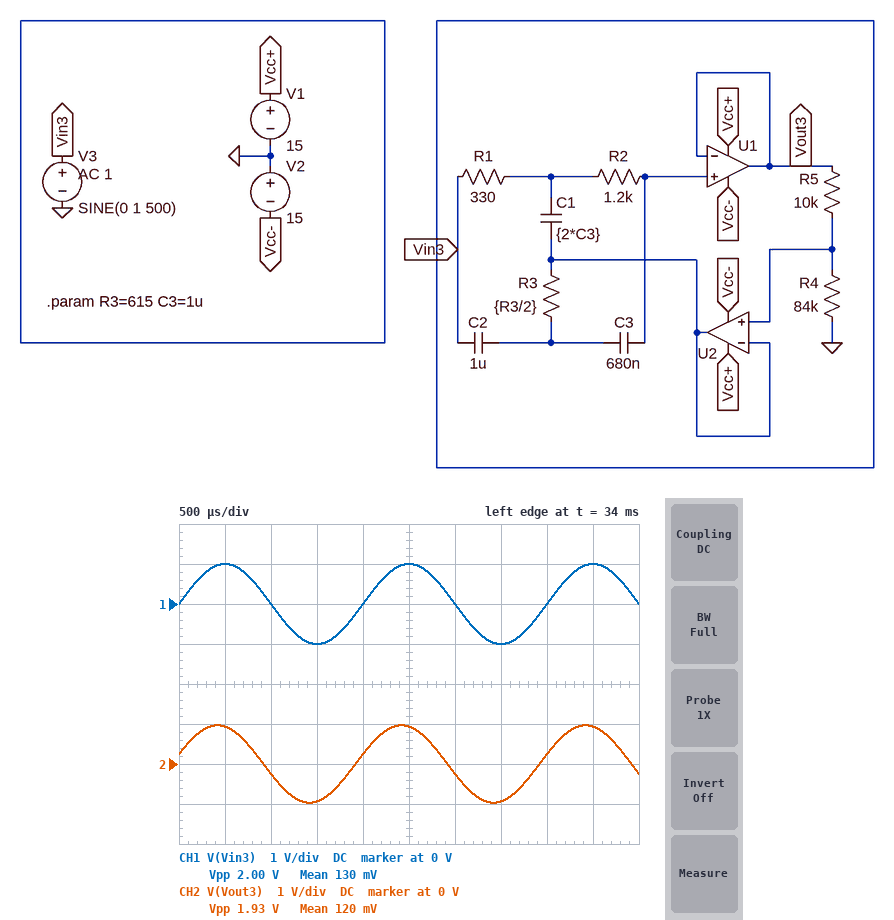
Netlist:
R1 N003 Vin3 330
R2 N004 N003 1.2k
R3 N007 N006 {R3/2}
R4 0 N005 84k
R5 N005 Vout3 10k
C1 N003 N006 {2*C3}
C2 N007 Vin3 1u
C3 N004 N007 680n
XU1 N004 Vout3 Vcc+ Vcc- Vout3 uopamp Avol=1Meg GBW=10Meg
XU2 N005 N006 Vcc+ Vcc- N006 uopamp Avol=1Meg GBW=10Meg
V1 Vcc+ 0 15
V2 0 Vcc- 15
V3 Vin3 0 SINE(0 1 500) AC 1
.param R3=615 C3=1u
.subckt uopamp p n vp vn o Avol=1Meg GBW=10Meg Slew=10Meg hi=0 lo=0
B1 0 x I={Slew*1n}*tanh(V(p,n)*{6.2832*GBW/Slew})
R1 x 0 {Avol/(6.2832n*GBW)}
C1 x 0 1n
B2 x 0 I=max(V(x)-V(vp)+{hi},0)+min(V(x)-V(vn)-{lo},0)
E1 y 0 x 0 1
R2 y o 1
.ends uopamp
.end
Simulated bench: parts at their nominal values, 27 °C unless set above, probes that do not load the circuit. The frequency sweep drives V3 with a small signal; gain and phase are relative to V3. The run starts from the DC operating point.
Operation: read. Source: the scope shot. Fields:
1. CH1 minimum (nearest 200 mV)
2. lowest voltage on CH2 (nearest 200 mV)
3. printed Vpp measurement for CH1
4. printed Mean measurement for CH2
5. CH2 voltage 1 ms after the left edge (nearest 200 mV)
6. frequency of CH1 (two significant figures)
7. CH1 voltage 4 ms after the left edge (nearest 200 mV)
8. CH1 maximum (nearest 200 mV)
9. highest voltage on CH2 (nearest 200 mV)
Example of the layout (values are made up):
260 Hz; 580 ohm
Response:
-1.0 V; -1.0 V; 2.00 V; 120 mV; -200 mV; 500 Hz; 0 V; 1.0 V; 1.0 V
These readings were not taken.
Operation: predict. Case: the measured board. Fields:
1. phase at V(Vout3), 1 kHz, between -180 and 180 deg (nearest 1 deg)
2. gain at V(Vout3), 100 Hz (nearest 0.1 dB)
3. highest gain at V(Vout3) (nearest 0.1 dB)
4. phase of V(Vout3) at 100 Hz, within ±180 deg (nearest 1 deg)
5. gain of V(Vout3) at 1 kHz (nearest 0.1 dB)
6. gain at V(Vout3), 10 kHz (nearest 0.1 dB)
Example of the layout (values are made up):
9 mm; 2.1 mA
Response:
6 deg; -0.1 dB; 0 dB; -7 deg; 0 dB; 0 dB
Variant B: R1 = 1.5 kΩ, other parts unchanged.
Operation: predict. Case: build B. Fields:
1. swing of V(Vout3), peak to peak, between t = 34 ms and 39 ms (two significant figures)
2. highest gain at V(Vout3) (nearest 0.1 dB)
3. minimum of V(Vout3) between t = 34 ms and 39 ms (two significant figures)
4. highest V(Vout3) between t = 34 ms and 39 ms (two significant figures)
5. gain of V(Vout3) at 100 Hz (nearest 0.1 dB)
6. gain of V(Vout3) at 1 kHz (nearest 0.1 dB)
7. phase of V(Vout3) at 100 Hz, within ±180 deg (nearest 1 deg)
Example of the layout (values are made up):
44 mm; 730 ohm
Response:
2.0 V; 7.2 dB; -1.0 V; 1.0 V; 0.3 dB; 0 dB; -27 deg
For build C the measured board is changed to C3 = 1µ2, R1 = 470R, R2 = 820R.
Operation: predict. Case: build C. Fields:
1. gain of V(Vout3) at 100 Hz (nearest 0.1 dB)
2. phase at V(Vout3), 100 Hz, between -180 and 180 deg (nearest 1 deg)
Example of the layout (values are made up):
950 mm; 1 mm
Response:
-0.2 dB; -11 deg
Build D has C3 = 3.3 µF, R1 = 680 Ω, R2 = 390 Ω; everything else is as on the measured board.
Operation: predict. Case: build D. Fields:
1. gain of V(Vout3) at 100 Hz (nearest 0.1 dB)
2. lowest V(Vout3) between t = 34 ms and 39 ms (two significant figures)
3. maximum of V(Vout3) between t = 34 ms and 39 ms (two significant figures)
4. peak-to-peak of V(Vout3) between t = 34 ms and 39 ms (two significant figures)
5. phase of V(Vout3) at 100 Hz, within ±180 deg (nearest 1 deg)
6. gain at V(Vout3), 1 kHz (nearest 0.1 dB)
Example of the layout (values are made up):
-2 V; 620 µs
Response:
-1.8 dB; -920 mV; 920 mV; 1.8 V; -17 deg; -0.2 dB
